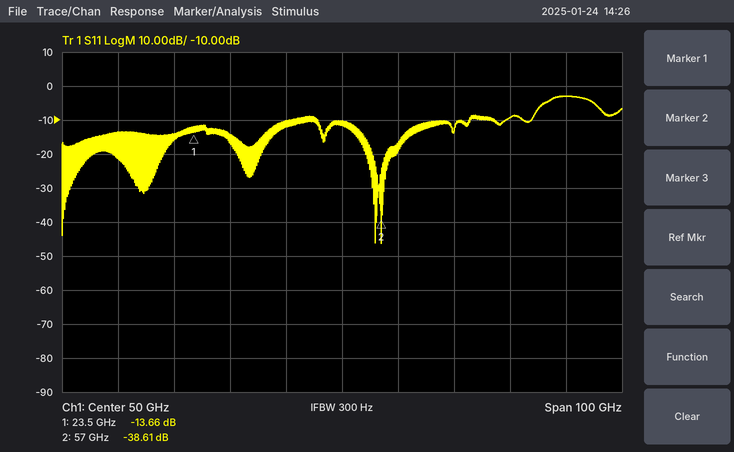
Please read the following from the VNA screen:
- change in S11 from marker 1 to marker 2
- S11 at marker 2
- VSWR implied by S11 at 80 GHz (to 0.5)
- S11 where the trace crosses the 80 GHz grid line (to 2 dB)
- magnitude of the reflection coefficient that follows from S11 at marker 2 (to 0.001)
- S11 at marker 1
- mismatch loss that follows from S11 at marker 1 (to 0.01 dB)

-24.95 dB
-38.61 dB
2.0
-10 dB
0.012
-13.66 dB
0.19 dB
